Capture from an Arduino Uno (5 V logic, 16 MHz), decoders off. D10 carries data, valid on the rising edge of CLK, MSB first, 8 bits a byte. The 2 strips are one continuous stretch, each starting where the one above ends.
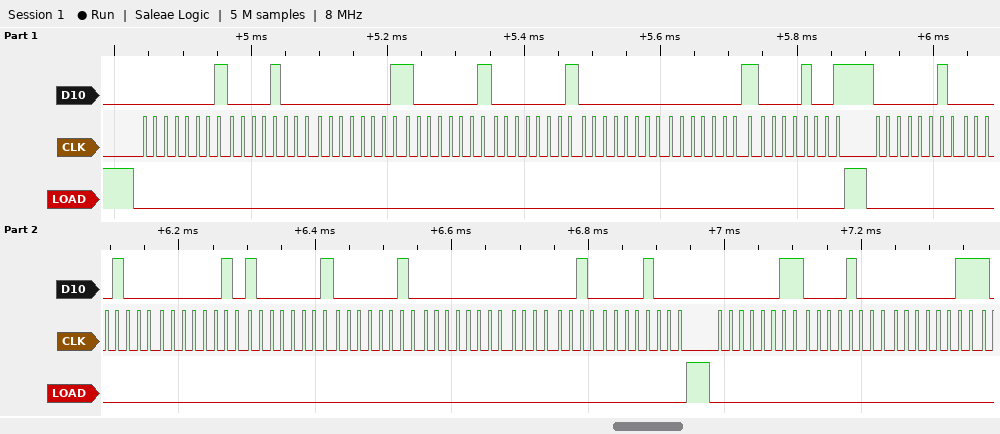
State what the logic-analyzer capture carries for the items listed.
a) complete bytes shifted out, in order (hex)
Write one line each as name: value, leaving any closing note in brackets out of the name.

complete bytes shifted out, in order: 01 08 01 81 01 00 01 09 02 08 02 81 02 00 02 08 03 08 03
